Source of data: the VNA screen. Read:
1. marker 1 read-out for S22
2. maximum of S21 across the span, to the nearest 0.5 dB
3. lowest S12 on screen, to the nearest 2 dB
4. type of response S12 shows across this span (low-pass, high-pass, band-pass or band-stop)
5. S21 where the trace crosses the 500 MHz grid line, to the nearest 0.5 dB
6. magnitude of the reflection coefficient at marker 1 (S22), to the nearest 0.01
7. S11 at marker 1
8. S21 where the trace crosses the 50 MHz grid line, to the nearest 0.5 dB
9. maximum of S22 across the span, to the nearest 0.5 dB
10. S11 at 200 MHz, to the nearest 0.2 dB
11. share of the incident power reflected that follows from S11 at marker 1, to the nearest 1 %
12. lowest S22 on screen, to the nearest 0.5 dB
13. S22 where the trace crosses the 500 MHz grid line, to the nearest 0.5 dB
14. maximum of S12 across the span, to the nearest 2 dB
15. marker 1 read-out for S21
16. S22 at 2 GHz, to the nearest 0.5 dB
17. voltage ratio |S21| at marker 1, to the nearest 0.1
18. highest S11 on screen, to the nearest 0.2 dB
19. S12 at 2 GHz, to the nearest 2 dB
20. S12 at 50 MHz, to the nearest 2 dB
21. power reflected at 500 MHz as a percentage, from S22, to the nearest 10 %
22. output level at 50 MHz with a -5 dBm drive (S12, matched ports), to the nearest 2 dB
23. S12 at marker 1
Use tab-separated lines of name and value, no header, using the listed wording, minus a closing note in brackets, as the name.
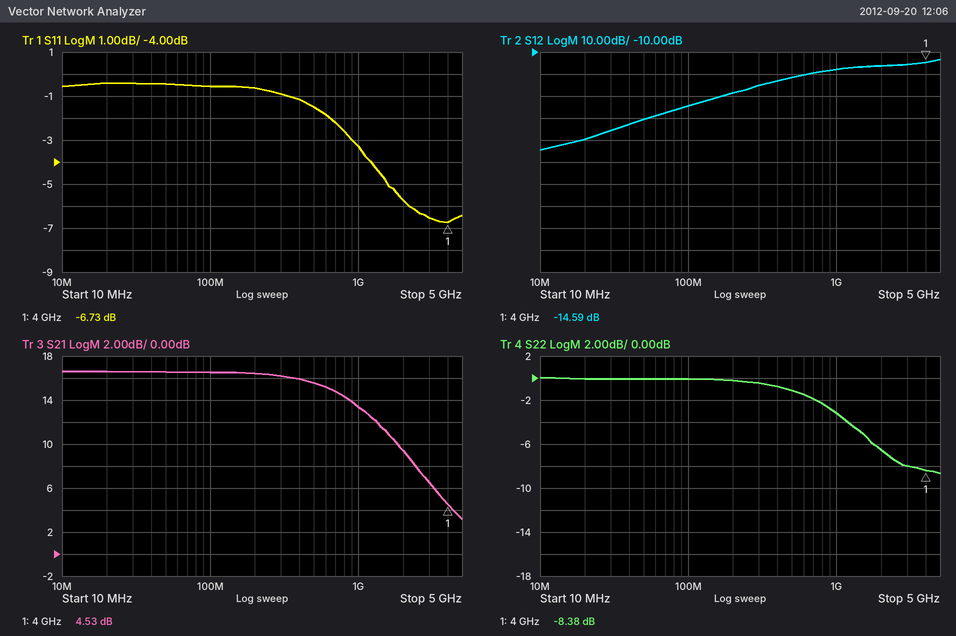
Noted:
marker 1 read-out for S22	-8.38 dB
maximum of S21 across the span, to the nearest 0.5 dB	16.5 dB
lowest S12 on screen, to the nearest 2 dB	-54 dB
type of response S12 shows across this span	high-pass
S21 where the trace crosses the 500 MHz grid line, to the nearest 0.5 dB	15.5 dB
magnitude of the reflection coefficient at marker 1 (S22), to the nearest 0.01	0.38
S11 at marker 1	-6.73 dB
S21 where the trace crosses the 50 MHz grid line, to the nearest 0.5 dB	16.5 dB
maximum of S22 across the span, to the nearest 0.5 dB	0.0 dB
S11 at 200 MHz, to the nearest 0.2 dB	-0.6 dB
share of the incident power reflected that follows from S11 at marker 1, to the nearest 1 %	21 %
lowest S22 on screen, to the nearest 0.5 dB	-8.5 dB
S22 where the trace crosses the 500 MHz grid line, to the nearest 0.5 dB	-1.0 dB
maximum of S12 across the span, to the nearest 2 dB	-14 dB
marker 1 read-out for S21	4.53 dB
S22 at 2 GHz, to the nearest 0.5 dB	-6.5 dB
voltage ratio |S21| at marker 1, to the nearest 0.1	1.7
highest S11 on screen, to the nearest 0.2 dB	-0.4 dB
S12 at 2 GHz, to the nearest 2 dB	-16 dB
S12 at 50 MHz, to the nearest 2 dB	-40 dB
power reflected at 500 MHz as a percentage, from S22, to the nearest 10 %	80 %
output level at 50 MHz with a -5 dBm drive (S12, matched ports), to the nearest 2 dB	-46 dBm
S12 at marker 1	-14.59 dB
